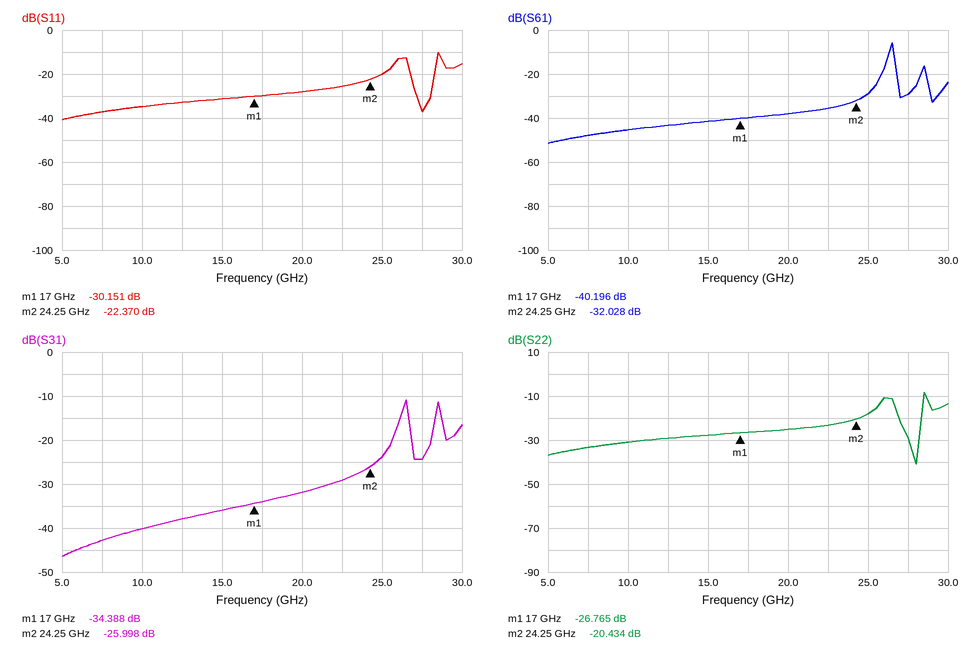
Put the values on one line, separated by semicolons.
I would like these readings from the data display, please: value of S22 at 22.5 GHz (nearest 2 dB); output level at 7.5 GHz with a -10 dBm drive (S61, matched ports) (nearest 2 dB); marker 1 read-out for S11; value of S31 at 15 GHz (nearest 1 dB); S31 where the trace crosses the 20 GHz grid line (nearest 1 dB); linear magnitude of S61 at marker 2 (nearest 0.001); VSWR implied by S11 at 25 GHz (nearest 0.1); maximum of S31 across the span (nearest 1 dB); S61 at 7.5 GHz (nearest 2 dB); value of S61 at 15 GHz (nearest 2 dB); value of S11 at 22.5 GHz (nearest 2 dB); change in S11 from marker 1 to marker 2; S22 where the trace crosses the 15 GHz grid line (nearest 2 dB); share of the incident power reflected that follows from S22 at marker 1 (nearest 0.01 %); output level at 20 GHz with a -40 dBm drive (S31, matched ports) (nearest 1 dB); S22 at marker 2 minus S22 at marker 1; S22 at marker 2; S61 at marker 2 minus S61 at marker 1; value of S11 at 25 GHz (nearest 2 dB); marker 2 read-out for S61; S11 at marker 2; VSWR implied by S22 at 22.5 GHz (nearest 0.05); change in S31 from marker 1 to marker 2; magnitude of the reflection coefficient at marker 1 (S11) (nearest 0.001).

-24 dB; -58 dBm; -30.151 dB; -36 dB; -32 dB; 0.025; 1.2; -11 dB; -48 dB; -42 dB; -26 dB; 7.781 dB; -28 dB; 0.21 %; -72 dBm; 6.331 dB; -20.434 dB; 8.168 dB; -20 dB; -32.028 dB; -22.370 dB; 1.15; 8.390 dB; 0.031
